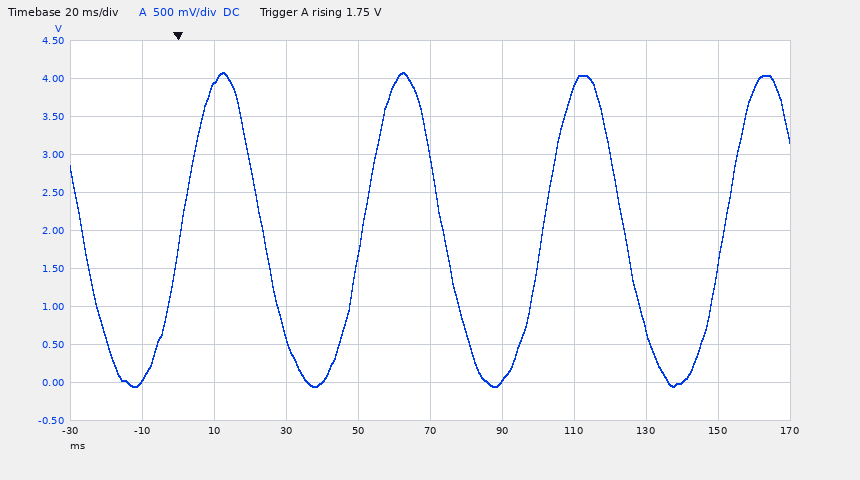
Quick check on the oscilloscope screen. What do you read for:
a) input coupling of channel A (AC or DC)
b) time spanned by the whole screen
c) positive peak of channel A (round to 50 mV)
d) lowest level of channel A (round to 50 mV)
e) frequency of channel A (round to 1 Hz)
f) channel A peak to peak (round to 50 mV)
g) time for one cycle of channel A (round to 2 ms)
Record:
DC
200 ms
4.10 V
-50 mV
20 Hz
4.15 V
50 ms
